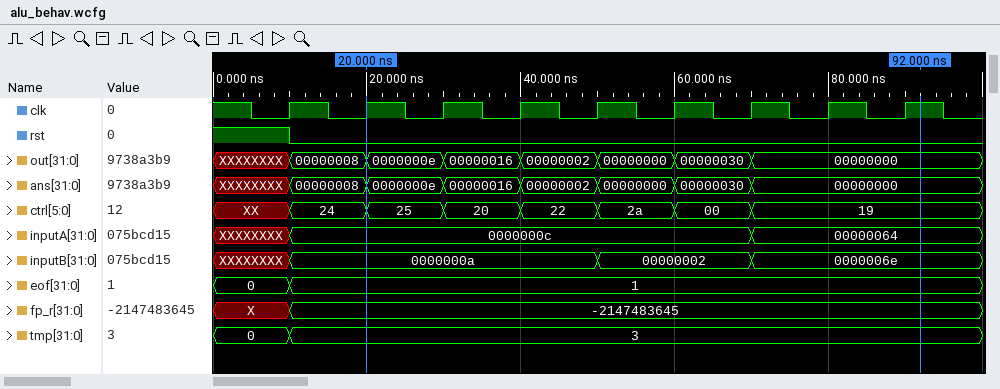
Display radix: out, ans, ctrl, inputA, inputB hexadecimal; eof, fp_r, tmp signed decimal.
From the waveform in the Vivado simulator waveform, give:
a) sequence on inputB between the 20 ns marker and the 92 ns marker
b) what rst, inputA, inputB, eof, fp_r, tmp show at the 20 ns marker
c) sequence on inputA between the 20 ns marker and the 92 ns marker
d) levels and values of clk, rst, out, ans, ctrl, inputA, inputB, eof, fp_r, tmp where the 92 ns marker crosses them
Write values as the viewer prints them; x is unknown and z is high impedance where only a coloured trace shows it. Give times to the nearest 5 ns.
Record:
0000000a, 00000002, 0000006e
rst=0, inputA=0000000c, inputB=0000000a, eof=1, fp_r=-2147483645, tmp=3
0000000c, 00000064
clk=1, rst=0, out=00000000, ans=00000000, ctrl=19, inputA=00000064, inputB=0000006e, eof=1, fp_r=-2147483645, tmp=3
